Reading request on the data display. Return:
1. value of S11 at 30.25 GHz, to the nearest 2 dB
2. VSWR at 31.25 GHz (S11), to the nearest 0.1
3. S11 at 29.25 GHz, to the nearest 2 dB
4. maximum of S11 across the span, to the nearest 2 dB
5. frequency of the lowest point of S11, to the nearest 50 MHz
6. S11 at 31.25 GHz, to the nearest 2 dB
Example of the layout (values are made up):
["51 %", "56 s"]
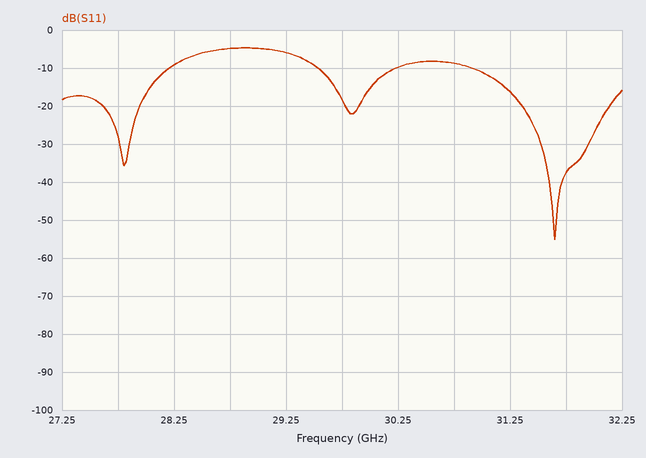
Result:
["-10 dB", "1.4", "-6 dB", "-4 dB", "31.65 GHz", "-16 dB"]
